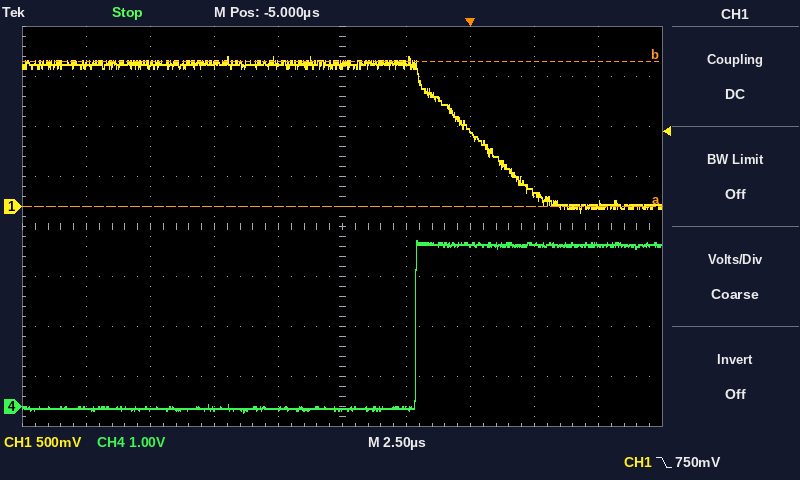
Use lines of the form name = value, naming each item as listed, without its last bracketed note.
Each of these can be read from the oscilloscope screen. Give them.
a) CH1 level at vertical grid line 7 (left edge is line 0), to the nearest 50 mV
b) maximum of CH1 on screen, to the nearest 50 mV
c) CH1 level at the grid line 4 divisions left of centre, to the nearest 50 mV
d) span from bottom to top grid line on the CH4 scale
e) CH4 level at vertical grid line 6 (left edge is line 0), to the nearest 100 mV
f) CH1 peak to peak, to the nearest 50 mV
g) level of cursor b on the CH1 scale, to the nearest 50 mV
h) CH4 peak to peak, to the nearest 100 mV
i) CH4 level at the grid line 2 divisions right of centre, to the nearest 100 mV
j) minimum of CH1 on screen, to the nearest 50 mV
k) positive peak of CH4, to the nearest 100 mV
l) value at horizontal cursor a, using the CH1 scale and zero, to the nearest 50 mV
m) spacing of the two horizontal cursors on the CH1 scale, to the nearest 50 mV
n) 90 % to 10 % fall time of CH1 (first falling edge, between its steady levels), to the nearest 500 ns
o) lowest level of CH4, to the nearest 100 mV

CH1 level at vertical grid line 7 (left edge is line 0), to the nearest 50 mV = 750 mV
maximum of CH1 on screen, to the nearest 50 mV = 1.50 V
CH1 level at the grid line 4 divisions left of centre, to the nearest 50 mV = 1.40 V
span from bottom to top grid line on the CH4 scale = 8 V
CH4 level at vertical grid line 6 (left edge is line 0), to the nearest 100 mV = 0.0 V
CH1 peak to peak, to the nearest 50 mV = 1.55 V
level of cursor b on the CH1 scale, to the nearest 50 mV = 1.45 V
CH4 peak to peak, to the nearest 100 mV = 3.4 V
CH4 level at the grid line 2 divisions right of centre, to the nearest 100 mV = 3.2 V
minimum of CH1 on screen, to the nearest 50 mV = -50 mV
positive peak of CH4, to the nearest 100 mV = 3.3 V
value at horizontal cursor a, using the CH1 scale and zero, to the nearest 50 mV = 0 mV
spacing of the two horizontal cursors on the CH1 scale, to the nearest 50 mV = 1.45 V
90 % to 10 % fall time of CH1 (first falling edge, between its steady levels), to the nearest 500 ns = 4.5 µs
lowest level of CH4, to the nearest 100 mV = -100 mV
